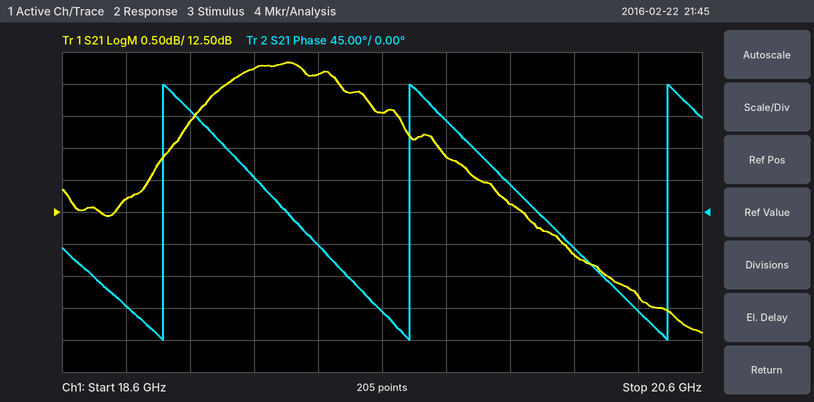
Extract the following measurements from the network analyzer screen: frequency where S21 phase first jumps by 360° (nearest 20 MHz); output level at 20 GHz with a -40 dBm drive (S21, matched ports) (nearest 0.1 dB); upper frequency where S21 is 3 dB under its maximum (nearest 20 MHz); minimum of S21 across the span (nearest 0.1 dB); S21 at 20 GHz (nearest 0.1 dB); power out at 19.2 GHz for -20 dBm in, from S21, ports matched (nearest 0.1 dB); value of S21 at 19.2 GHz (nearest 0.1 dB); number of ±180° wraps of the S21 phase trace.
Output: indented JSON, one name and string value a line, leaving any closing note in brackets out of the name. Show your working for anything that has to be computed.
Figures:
{
  "frequency where S21 phase first jumps by 360°": "18.92 GHz",
  "output level at 20 GHz with a -40 dBm drive (S21, matched ports)": "-40 dBm + (12.6 dB) = -27.4 dBm",
  "upper frequency where S21 is 3 dB under its maximum": "20.20 GHz",
  "minimum of S21 across the span": "10.6 dB",
  "S21 at 20 GHz": "12.6 dB",
  "power out at 19.2 GHz for -20 dBm in, from S21, ports matched": "-20 dBm + (14.7 dB) = -5.3 dBm",
  "value of S21 at 19.2 GHz": "14.7 dB",
  "number of ±180° wraps of the S21 phase trace": "3"
}
